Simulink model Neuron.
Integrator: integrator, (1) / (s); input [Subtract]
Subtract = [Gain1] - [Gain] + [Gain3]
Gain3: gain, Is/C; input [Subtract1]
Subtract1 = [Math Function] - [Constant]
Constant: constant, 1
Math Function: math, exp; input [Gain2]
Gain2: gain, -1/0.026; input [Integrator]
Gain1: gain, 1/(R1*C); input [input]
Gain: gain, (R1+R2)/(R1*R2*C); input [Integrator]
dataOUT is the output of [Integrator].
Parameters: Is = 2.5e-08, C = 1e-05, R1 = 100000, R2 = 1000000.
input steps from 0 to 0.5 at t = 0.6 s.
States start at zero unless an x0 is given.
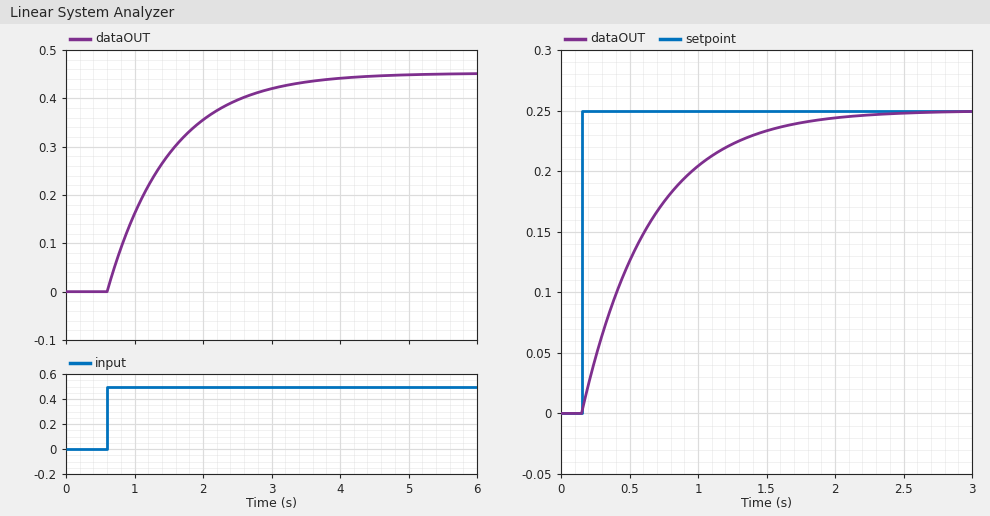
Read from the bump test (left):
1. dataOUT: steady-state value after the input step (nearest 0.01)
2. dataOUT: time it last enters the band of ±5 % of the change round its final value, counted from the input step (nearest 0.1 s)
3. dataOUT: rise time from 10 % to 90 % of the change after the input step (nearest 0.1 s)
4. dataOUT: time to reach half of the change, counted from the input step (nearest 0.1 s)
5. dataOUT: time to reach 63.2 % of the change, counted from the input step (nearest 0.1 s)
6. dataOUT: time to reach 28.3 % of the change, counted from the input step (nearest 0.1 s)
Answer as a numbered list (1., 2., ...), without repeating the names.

1. 0.45
2. 2.7 s
3. 2.0 s
4. 0.6 s
5. 0.9 s
6. 0.3 s
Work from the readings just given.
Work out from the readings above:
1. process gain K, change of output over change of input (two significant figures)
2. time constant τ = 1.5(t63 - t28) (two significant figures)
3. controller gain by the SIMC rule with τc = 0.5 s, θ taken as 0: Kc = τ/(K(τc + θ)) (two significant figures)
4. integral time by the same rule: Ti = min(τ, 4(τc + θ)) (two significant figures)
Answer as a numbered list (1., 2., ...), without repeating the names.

1. 0.90
2. 0.90 s
3. 2.0
4. 0.90 s
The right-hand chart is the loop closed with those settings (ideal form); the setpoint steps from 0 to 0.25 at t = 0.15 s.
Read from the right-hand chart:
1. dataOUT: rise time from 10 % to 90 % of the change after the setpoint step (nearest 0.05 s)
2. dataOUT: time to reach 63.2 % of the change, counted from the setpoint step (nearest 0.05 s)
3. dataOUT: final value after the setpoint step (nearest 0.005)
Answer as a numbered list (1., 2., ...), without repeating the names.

1. 1.10 s
2. 0.50 s
3. 0.250
